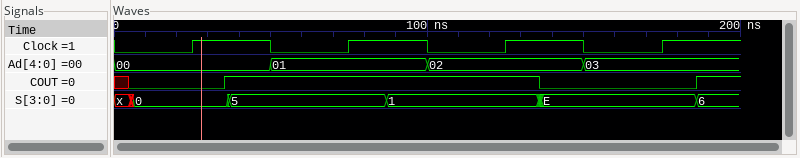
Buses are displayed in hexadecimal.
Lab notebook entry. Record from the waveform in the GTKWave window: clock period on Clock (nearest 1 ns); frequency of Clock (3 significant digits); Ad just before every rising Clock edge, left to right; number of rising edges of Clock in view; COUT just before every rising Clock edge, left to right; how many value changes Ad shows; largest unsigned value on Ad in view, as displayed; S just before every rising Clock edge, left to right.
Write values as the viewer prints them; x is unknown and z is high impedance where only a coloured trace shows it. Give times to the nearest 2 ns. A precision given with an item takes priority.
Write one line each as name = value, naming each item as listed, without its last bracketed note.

clock period on Clock = 50 ns
frequency of Clock = 20.0 MHz
Ad just before every rising Clock edge, left to right = 00, 01, 02, 03
number of rising edges of Clock in view = 4
COUT just before every rising Clock edge, left to right = 0 1 1 0
how many value changes Ad shows = 3
largest unsigned value on Ad in view, as displayed = 03
S just before every rising Clock edge, left to right = 0, 5, 1, E
